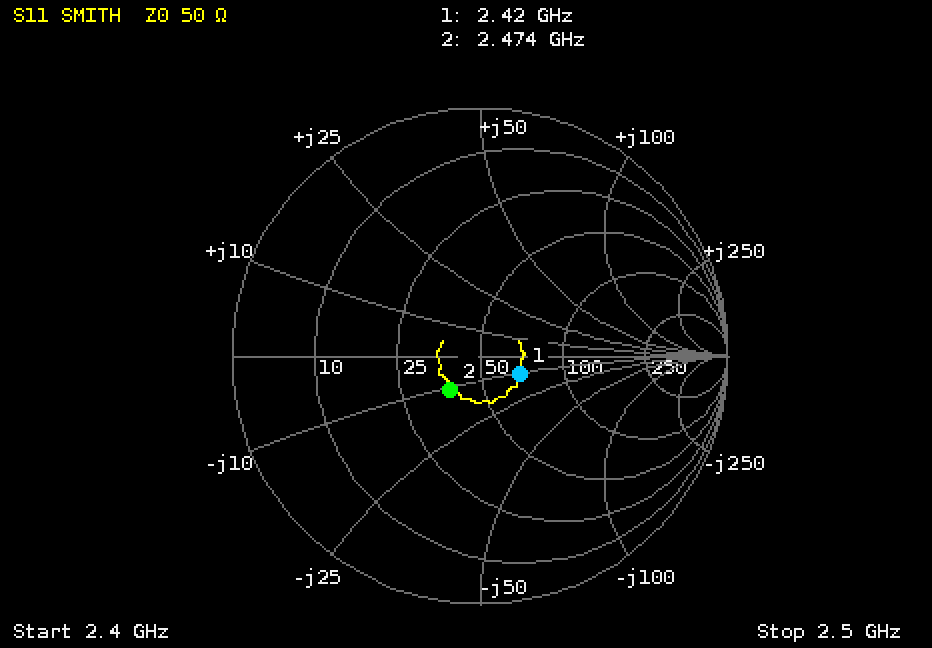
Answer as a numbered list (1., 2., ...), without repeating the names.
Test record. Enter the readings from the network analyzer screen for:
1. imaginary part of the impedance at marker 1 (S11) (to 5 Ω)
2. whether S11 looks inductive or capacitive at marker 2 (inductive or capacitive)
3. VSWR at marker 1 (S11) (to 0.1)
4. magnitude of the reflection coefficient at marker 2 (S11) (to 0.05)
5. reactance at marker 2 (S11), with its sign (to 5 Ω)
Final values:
1. -10 Ω
2. capacitive
3. 1.4
4. 0.20
5. -10 Ω
